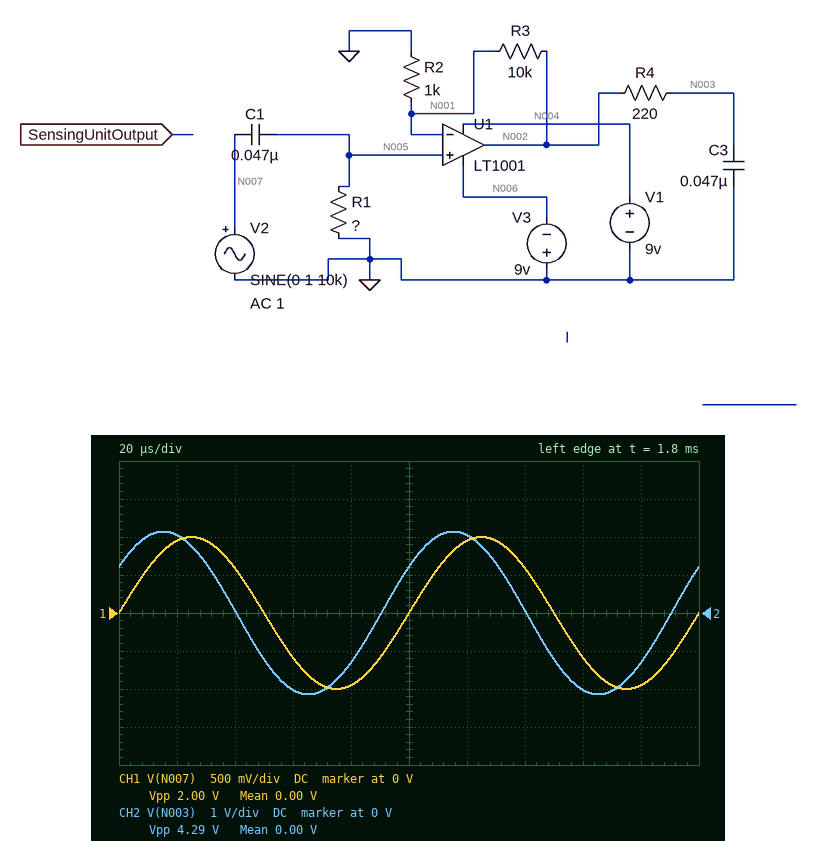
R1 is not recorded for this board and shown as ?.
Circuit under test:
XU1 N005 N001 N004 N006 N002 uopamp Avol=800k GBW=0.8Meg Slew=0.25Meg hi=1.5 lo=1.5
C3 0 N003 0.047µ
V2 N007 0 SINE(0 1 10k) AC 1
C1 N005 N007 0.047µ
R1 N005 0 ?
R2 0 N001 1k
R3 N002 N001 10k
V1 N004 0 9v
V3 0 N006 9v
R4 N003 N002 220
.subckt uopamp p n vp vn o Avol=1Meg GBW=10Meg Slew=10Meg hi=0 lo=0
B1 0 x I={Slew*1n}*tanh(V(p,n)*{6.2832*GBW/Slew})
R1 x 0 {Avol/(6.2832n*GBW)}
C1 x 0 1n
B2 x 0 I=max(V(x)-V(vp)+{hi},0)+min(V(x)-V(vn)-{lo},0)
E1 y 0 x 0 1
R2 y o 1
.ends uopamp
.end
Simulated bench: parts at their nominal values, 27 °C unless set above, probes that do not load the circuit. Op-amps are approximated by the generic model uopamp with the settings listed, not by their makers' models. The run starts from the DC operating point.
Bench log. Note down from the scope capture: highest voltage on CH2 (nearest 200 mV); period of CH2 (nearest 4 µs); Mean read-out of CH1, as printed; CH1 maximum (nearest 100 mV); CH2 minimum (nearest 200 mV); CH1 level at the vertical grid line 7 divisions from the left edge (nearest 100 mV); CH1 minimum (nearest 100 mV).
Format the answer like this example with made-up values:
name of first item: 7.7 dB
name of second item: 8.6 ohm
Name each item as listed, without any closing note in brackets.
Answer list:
highest voltage on CH2: 2.2 V
period of CH2: 100 µs
Mean read-out of CH1, as printed: 0.00 V
CH1 maximum: 1.0 V
CH2 minimum: -2.2 V
CH1 level at the vertical grid line 7 divisions from the left edge: 600 mV
CH1 minimum: -1.0 V
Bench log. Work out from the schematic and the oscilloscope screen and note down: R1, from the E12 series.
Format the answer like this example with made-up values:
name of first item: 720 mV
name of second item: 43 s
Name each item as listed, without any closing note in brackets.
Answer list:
R1, from the E12 series: 82 Ω
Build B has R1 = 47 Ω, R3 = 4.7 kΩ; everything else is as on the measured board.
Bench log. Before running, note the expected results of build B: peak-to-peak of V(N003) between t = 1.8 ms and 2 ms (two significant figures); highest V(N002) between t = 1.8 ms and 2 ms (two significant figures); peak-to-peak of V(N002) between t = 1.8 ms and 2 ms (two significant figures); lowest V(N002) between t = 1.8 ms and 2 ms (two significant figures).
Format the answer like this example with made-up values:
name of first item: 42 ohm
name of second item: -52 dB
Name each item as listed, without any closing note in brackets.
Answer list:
peak-to-peak of V(N003) between t = 1.8 ms and 2 ms: 1.3 V
highest V(N002) between t = 1.8 ms and 2 ms: 780 mV
peak-to-peak of V(N002) between t = 1.8 ms and 2 ms: 1.6 V
lowest V(N002) between t = 1.8 ms and 2 ms: -780 mV
